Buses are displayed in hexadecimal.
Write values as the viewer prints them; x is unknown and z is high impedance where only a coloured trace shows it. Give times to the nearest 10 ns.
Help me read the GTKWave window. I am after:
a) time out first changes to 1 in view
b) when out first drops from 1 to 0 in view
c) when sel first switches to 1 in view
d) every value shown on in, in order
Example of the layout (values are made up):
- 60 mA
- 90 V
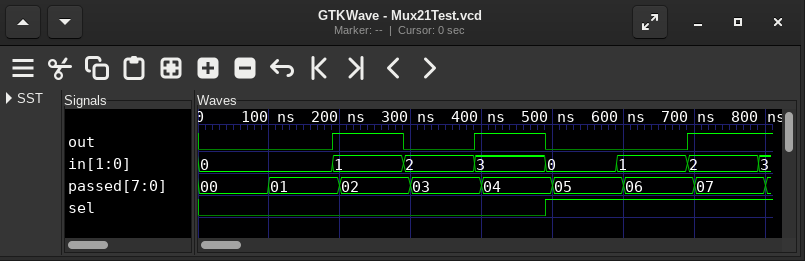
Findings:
- 190 ns
- 290 ns
- 490 ns
- 0, 1, 2, 3, 0, 1, 2, 3
